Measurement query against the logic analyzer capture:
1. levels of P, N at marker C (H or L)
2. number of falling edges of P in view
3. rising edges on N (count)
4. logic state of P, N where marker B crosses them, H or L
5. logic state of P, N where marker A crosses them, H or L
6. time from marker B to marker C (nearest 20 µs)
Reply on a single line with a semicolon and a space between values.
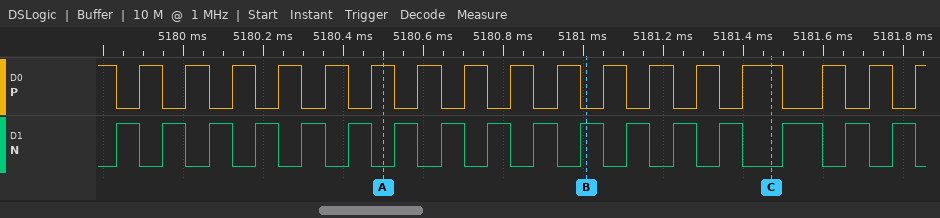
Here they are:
P=H, N=L; 17; 17; P=L, N=H; P=H, N=L; 460 µs
